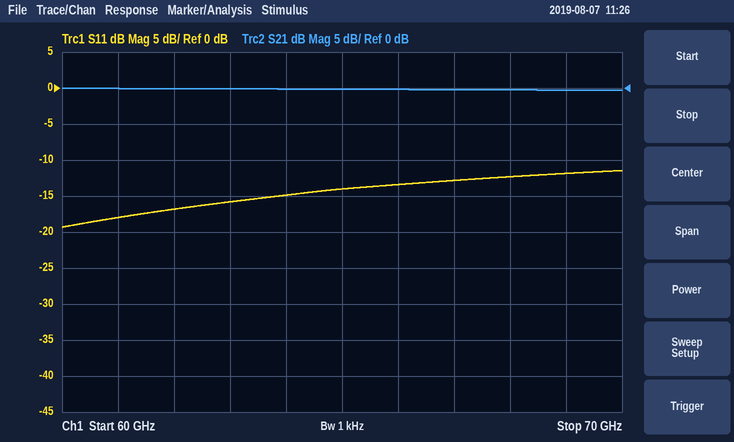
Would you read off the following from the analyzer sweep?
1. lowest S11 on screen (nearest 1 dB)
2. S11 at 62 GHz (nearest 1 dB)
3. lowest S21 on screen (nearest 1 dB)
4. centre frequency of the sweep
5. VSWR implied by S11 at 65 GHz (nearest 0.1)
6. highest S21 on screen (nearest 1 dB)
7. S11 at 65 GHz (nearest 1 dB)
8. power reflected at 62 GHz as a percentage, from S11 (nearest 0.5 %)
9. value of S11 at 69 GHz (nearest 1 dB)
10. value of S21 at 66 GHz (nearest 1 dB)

-19 dB
-17 dB
0 dB
65 GHz
1.5
0 dB
-14 dB
2.0 %
-12 dB
0 dB
